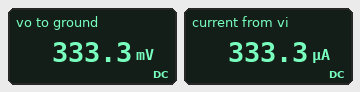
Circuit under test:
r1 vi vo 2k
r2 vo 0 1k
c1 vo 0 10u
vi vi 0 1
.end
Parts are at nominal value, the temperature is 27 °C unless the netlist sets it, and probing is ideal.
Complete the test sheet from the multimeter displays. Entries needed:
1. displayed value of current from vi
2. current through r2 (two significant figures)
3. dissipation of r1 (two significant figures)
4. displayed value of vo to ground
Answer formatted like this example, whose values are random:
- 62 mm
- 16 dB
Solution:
- 333.3 µA
- 330 µA
- 220 µW
- 333.3 mV
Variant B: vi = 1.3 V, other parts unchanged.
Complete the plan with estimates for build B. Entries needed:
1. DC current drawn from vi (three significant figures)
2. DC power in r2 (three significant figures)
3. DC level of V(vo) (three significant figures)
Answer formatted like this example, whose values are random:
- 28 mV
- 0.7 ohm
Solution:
- 433 µA
- 188 µW
- 433 mV
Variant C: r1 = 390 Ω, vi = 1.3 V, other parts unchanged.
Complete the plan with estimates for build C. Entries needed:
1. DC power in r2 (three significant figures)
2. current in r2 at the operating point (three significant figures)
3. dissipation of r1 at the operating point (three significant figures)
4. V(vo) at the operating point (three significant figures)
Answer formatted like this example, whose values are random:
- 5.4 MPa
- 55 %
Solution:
- 875 µW
- 935 µA
- 341 µW
- 935 mV
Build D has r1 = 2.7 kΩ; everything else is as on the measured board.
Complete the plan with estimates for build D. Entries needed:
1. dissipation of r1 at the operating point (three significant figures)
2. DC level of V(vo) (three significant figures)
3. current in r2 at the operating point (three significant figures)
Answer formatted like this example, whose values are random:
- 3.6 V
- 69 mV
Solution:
- 197 µW
- 270 mV
- 270 µA
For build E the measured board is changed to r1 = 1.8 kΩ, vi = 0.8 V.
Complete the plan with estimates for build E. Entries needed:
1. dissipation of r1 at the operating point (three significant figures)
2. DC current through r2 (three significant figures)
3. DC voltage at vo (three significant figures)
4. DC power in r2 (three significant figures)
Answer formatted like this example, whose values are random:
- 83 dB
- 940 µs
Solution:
- 147 µW
- 286 µA
- 286 mV
- 81.6 µW
